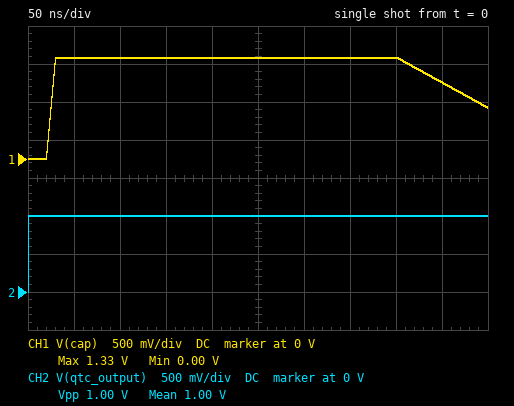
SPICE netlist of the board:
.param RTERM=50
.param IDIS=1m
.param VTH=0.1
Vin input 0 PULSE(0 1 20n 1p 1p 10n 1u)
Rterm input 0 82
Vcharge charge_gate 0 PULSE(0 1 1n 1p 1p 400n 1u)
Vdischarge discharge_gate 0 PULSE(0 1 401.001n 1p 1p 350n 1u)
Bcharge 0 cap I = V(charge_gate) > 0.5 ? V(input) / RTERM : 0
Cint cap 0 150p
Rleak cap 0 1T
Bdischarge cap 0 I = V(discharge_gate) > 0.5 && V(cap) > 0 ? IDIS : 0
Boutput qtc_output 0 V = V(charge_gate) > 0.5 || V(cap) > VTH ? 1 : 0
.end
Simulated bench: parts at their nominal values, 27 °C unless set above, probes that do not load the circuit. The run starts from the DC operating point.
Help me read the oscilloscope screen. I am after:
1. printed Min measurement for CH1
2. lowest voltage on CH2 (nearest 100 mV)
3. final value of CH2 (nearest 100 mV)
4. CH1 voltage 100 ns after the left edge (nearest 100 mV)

0.00 V
0 V
1.0 V
1.3 V
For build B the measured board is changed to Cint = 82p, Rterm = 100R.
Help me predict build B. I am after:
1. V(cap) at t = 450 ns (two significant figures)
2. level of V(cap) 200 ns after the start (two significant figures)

1.8 V
2.4 V
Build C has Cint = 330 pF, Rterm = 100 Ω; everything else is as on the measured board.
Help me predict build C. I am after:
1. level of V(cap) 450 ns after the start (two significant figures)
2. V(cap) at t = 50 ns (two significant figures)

460 mV
610 mV
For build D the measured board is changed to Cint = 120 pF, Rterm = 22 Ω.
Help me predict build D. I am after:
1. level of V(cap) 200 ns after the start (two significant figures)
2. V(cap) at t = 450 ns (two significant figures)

1.7 V
1.3 V
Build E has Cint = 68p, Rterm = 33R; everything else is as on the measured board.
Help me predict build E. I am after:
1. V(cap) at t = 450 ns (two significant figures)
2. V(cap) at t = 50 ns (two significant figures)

2.2 V
2.9 V
